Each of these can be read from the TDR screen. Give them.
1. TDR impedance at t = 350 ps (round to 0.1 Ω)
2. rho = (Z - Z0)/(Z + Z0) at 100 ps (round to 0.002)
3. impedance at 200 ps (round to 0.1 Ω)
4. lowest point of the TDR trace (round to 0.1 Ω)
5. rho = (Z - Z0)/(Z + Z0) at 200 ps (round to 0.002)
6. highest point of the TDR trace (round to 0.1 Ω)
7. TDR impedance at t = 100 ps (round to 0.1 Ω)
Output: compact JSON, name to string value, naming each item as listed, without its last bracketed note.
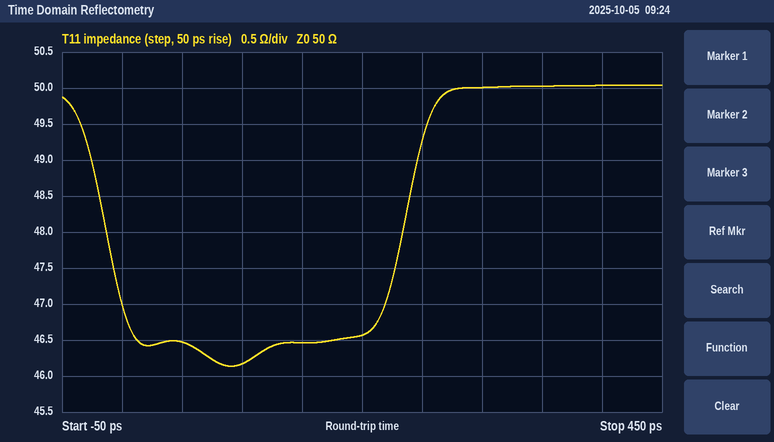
{"TDR impedance at t = 350 ps": "50.0 Ω", "rho = (Z - Z0)/(Z + Z0) at 100 ps": "-0.040", "impedance at 200 ps": "46.6 Ω", "lowest point of the TDR trace": "46.1 Ω", "rho = (Z - Z0)/(Z + Z0) at 200 ps": "-0.036", "highest point of the TDR trace": "50.0 Ω", "TDR impedance at t = 100 ps": "46.2 Ω"}
